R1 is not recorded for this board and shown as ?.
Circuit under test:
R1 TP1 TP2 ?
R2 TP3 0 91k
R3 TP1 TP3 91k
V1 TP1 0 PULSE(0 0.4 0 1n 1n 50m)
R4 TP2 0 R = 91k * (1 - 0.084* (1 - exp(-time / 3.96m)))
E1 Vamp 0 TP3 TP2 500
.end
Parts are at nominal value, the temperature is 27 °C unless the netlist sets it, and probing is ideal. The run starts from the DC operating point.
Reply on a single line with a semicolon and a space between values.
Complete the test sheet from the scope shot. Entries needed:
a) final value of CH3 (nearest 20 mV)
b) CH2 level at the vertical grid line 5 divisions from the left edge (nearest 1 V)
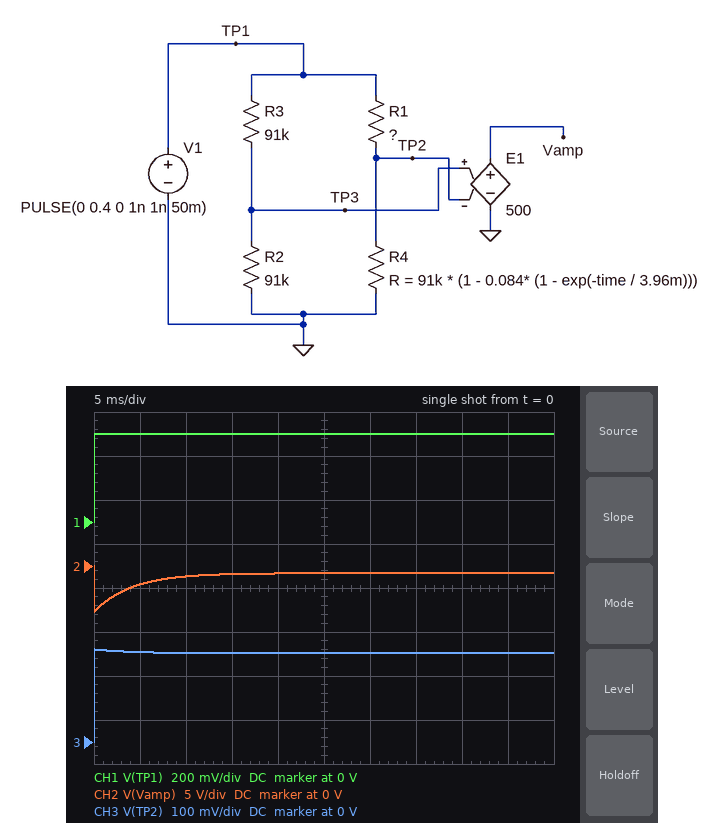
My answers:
200 mV; -1 V
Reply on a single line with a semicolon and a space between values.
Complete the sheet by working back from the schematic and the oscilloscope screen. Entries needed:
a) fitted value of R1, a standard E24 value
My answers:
82 kΩ
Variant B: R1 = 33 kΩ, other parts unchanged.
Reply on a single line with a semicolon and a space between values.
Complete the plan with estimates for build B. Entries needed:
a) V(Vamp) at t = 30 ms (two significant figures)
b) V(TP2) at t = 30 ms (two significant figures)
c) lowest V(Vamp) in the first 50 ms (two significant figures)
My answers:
-43 V; 290 mV; -47 V
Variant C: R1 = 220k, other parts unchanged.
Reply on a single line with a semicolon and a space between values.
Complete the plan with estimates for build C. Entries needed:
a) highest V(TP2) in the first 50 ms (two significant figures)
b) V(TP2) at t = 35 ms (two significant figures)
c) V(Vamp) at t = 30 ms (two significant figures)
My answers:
120 mV; 110 mV; 45 V
